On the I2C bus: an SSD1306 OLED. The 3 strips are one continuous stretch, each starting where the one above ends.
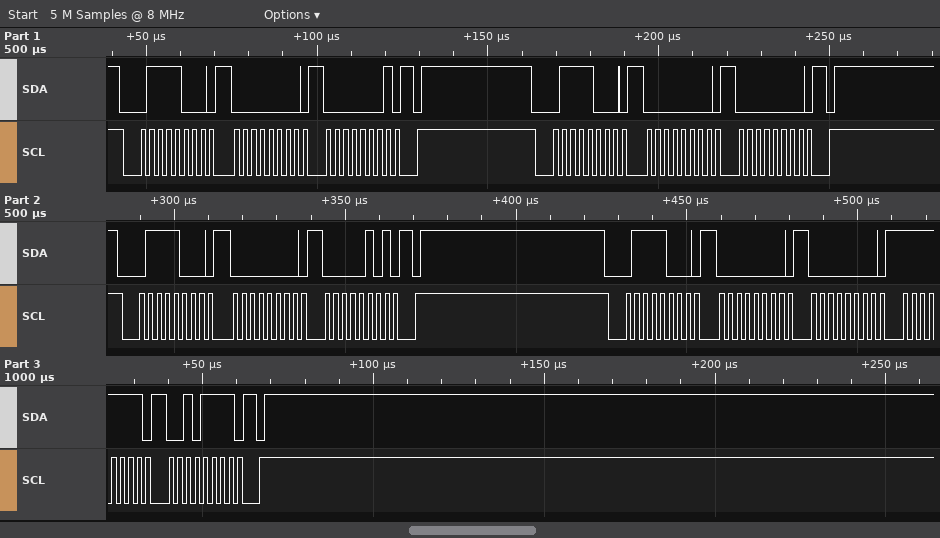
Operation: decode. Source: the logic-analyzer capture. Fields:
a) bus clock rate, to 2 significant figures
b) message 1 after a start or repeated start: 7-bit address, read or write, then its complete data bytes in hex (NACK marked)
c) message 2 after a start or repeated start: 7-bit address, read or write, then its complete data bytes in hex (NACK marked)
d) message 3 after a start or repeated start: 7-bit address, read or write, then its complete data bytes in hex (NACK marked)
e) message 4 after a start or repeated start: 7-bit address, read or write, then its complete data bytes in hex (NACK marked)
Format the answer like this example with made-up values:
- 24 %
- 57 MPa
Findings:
- 400 kHz
- 0x3C write: 00 01
- 0x3C write: 00 00
- 0x3C write: 00 05
- 0x3C write: 00 00 FF 2F
